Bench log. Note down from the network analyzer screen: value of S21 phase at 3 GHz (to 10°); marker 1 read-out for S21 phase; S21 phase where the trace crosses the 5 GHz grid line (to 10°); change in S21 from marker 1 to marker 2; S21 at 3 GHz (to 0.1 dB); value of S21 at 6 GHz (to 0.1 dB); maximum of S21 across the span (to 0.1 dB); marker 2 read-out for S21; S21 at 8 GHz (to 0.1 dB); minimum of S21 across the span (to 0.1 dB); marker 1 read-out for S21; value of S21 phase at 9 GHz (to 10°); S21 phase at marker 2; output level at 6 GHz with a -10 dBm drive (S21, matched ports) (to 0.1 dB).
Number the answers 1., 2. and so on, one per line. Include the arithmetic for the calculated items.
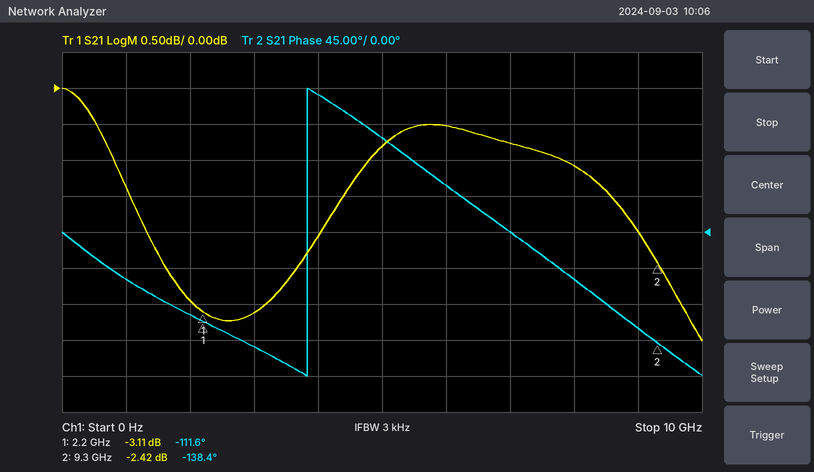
1. -140°
2. -111.6°
3. 120°
4. -2.42 − (-3.11) = 0.69 dB
5. -3.1 dB
6. -0.5 dB
7. 0.0 dB
8. -2.42 dB
9. -1.1 dB
10. -3.5 dB
11. -3.11 dB
12. -120°
13. -138.4°
14. -10 dBm + (-0.5 dB) = -10.5 dBm
